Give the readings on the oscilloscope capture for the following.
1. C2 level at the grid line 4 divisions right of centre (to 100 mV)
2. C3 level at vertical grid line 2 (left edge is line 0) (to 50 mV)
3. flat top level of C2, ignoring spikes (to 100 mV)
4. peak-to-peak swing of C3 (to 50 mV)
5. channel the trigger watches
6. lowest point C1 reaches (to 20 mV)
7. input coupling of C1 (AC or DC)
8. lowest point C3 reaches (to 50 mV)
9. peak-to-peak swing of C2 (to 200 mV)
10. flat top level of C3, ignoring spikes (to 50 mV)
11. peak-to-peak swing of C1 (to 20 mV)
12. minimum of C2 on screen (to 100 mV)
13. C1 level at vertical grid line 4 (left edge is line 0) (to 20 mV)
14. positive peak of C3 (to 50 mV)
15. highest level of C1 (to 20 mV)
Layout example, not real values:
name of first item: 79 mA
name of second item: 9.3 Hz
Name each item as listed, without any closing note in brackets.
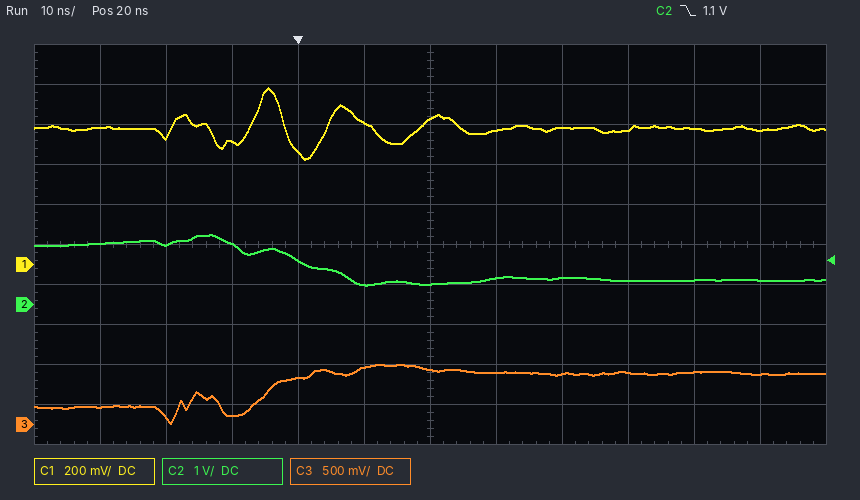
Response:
C2 level at the grid line 4 divisions right of centre: 600 mV
C3 level at vertical grid line 2 (left edge is line 0): 100 mV
flat top level of C2, ignoring spikes: 1.5 V
peak-to-peak swing of C3: 750 mV
channel the trigger watches: C2
lowest point C1 reaches: 520 mV
input coupling of C1: DC
lowest point C3 reaches: 0 mV
peak-to-peak swing of C2: 1.2 V
flat top level of C3, ignoring spikes: 650 mV
peak-to-peak swing of C1: 360 mV
minimum of C2 on screen: 500 mV
C1 level at vertical grid line 4 (left edge is line 0): 560 mV
positive peak of C3: 750 mV
highest level of C1: 880 mV
